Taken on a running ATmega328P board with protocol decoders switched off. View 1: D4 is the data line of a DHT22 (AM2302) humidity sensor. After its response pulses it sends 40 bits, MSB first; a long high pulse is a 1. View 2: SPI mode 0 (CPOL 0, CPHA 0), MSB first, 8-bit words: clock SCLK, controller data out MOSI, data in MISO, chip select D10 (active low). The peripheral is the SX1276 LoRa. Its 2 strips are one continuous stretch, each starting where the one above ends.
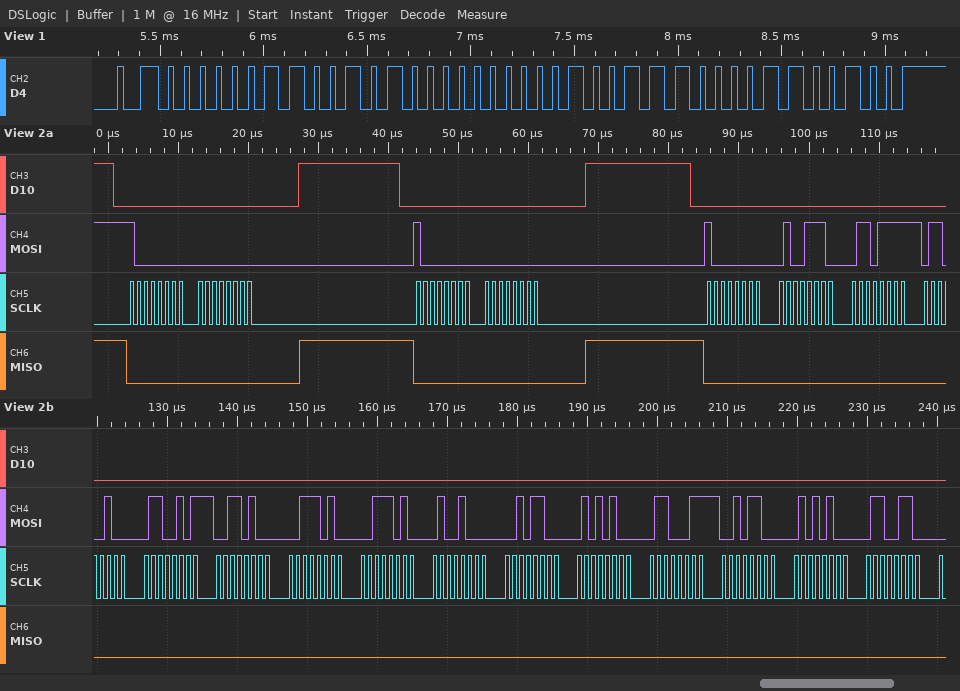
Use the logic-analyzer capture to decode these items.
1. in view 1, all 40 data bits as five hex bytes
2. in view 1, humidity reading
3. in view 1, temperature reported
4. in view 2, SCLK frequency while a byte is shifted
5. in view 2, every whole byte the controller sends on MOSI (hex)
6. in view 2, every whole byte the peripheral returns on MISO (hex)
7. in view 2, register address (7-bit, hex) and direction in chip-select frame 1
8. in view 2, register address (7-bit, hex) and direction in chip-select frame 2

03 28 01 38 64
80.8 %
31.2 °C
1 MHz
80 00 80 00 80 4E 6F 64 65 34 3A 3A 48 2C 54 63 2C 54 66
00 00 00 00 00 00 00 00 00 00 00 00 00 00 00 00 00 00 00
0x00 write
0x00 write
